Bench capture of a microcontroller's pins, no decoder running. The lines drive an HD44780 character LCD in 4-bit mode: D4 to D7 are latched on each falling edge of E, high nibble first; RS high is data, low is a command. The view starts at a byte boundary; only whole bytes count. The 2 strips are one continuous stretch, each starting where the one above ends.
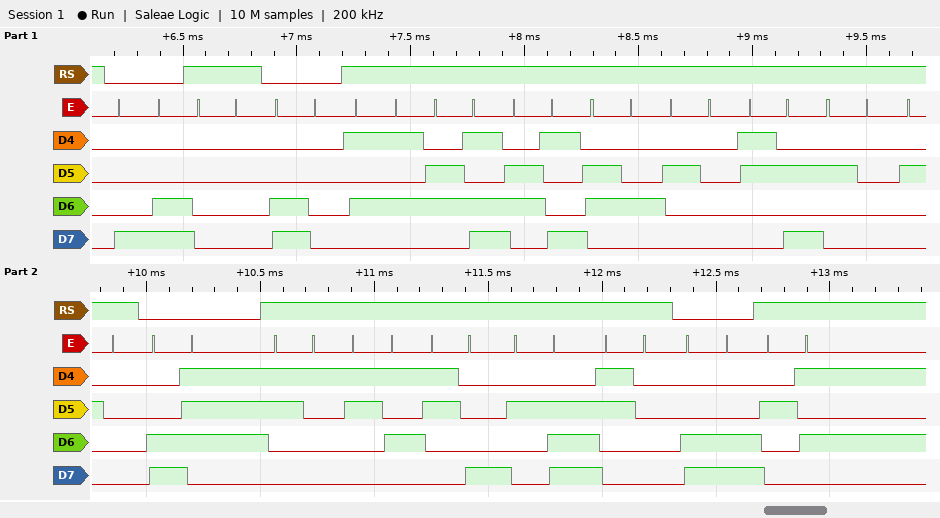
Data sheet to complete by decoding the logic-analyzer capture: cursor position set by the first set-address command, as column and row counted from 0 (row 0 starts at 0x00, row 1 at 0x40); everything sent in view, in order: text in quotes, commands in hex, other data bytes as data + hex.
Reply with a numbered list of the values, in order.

1. column 12, row 0
2. 0x8C data 00 0xC0 "Umid :  " 0xC7 "158.0" 0xCC "%"
